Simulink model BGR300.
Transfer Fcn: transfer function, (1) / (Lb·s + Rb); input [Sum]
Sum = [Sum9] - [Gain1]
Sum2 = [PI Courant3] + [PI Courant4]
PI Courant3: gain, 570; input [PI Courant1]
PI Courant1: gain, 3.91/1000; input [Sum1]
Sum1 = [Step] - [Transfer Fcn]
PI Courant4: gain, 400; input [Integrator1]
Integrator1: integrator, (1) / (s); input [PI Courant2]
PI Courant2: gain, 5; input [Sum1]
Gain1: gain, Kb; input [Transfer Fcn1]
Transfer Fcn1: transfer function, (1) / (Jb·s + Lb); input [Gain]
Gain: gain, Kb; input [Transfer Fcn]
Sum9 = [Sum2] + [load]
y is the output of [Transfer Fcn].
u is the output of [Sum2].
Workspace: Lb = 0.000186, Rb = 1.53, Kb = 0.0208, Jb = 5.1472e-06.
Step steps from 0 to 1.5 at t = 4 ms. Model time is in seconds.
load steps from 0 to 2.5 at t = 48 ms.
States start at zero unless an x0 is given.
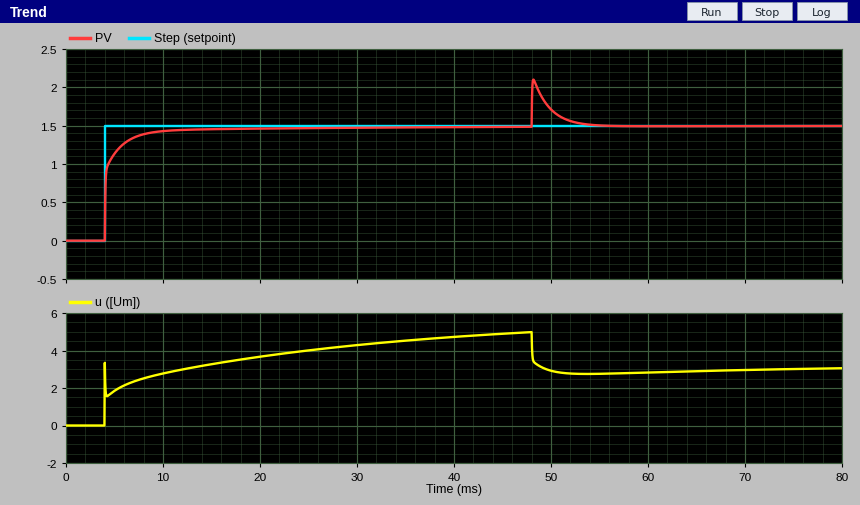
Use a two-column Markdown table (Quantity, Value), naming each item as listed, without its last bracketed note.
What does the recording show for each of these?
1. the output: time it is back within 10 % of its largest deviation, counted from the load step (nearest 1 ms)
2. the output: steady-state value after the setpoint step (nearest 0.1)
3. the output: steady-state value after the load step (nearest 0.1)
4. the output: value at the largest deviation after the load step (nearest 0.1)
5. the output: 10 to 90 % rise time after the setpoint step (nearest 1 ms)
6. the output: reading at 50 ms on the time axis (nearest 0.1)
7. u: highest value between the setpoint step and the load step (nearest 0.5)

| Quantity | Value |
|---|---|
| the output: time it is back within 10 % of its largest deviation, counted from the load step | 4 ms |
| the output: steady-state value after the setpoint step | 1.5 |
| the output: steady-state value after the load step | 1.5 |
| the output: value at the largest deviation after the load step | 2.1 |
| the output: 10 to 90 % rise time after the setpoint step | 3 ms |
| the output: reading at 50 ms on the time axis | 1.7 |
| u: highest value between the setpoint step and the load step | 5.0 |
